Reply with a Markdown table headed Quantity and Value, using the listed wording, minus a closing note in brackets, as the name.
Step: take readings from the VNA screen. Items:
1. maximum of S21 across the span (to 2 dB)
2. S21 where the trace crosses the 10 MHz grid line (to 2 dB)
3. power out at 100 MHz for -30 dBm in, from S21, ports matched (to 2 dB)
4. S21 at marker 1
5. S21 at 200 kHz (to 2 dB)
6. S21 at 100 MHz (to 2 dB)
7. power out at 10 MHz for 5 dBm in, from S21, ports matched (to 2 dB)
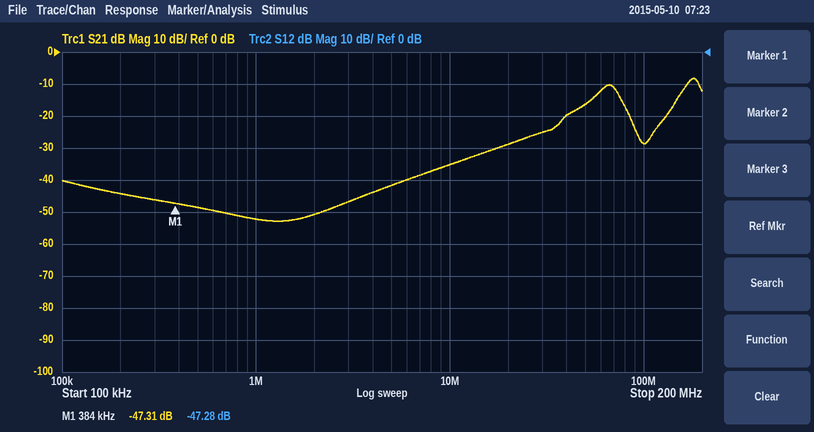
| Quantity | Value |
|---|---|
| maximum of S21 across the span | -8 dB |
| S21 where the trace crosses the 10 MHz grid line | -36 dB |
| power out at 100 MHz for -30 dBm in, from S21, ports matched | -58 dBm |
| S21 at marker 1 | -47.31 dB |
| S21 at 200 kHz | -44 dB |
| S21 at 100 MHz | -28 dB |
| power out at 10 MHz for 5 dBm in, from S21, ports matched | -30 dBm |
